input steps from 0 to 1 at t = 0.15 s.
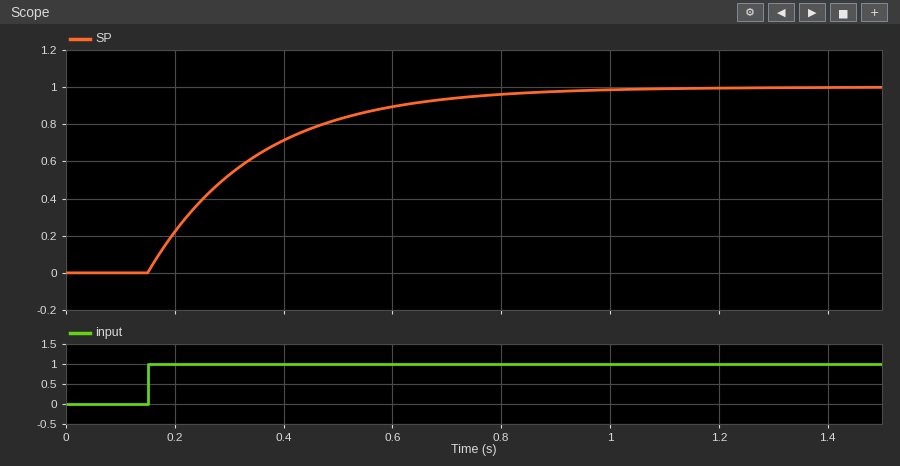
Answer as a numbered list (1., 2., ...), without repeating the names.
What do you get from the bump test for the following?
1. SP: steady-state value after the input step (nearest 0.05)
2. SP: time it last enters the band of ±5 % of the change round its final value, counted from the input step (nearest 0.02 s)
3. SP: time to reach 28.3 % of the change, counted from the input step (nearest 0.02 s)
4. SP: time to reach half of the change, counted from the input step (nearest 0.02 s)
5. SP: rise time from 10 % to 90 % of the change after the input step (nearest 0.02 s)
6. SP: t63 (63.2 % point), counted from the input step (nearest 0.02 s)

1. 1.00
2. 0.60 s
3. 0.06 s
4. 0.14 s
5. 0.44 s
6. 0.20 s
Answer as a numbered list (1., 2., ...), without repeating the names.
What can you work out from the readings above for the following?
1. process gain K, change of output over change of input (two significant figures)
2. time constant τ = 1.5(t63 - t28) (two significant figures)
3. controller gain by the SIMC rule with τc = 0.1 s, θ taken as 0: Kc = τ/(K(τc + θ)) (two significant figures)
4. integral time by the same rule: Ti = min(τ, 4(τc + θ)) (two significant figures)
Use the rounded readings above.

1. 1.0
2. 0.21 s
3. 2.1
4. 0.21 s
